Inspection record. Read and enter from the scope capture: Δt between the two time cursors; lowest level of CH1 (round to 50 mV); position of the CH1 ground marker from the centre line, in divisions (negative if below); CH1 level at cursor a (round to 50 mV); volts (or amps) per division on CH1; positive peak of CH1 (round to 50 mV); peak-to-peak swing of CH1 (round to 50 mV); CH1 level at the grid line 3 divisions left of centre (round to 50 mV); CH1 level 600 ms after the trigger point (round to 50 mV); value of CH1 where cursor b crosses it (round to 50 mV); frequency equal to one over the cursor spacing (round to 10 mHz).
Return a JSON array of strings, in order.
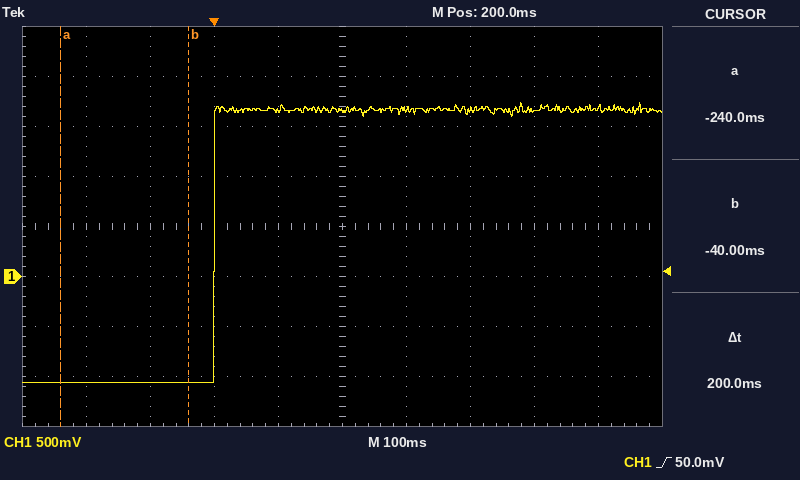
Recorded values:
["200 ms", "-1.05 V", "-1.0 div", "-1.05 V", "500 mV", "1.75 V", "2.80 V", "-1.05 V", "1.70 V", "-1.05 V", "5.00 Hz"]
